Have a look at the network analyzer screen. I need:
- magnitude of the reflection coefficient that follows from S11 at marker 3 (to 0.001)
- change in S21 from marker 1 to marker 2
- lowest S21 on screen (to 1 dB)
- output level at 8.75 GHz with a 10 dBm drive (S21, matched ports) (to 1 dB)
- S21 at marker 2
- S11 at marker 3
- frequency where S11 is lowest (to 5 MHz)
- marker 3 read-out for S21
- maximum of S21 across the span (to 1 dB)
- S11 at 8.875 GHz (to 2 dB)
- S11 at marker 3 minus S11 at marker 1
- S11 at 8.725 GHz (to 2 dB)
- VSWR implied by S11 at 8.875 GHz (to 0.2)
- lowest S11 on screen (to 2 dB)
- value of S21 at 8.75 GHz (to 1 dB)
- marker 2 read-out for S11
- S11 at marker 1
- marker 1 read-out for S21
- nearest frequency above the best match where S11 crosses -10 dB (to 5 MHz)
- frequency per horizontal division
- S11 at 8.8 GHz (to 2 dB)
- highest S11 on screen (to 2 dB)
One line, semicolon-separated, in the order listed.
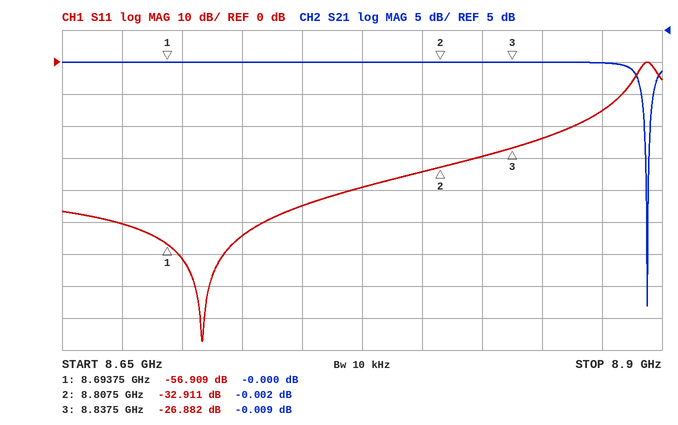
0.045; -0.002 dB; -38 dB; 10 dBm; -0.002 dB; -26.882 dB; 8.710 GHz; -0.009 dB; 0 dB; -16 dB; 30.027 dB; -54 dB; 1.4; -88 dB; 0 dB; -32.911 dB; -56.909 dB; -0.000 dB; 8.885 GHz; 25 MHz; -34 dB; 0 dB
